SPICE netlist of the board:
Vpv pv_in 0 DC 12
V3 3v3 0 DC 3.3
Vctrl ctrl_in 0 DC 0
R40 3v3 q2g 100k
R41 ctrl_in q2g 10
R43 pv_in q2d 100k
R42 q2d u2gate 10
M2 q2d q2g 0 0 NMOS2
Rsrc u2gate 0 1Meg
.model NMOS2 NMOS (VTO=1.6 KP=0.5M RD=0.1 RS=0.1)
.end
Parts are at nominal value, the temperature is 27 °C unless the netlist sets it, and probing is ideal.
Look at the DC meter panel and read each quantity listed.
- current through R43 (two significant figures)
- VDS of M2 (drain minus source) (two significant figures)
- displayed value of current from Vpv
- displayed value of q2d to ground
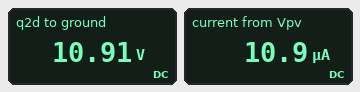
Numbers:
11 µA
11 V
10.9 µA
10.91 V
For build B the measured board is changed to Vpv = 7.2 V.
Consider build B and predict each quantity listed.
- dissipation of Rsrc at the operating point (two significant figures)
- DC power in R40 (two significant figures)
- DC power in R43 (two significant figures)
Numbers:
43 µW
110 µW
4.3 µW
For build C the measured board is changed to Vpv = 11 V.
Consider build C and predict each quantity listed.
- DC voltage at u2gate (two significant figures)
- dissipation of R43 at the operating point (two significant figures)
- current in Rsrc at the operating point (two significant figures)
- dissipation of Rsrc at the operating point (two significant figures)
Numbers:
10 V
10 µW
10 µA
100 µW
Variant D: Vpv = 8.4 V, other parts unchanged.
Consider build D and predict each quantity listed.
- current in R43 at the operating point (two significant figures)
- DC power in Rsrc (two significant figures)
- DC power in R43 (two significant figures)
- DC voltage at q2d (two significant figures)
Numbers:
7.6 µA
58 µW
5.8 µW
7.6 V
